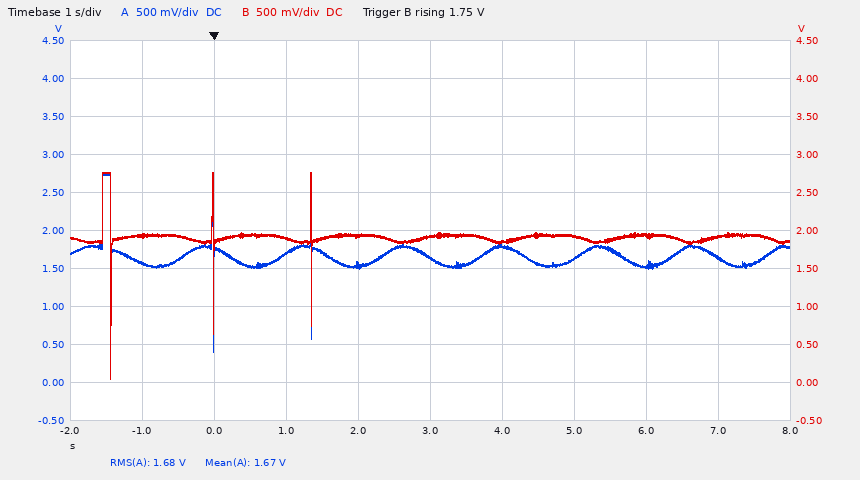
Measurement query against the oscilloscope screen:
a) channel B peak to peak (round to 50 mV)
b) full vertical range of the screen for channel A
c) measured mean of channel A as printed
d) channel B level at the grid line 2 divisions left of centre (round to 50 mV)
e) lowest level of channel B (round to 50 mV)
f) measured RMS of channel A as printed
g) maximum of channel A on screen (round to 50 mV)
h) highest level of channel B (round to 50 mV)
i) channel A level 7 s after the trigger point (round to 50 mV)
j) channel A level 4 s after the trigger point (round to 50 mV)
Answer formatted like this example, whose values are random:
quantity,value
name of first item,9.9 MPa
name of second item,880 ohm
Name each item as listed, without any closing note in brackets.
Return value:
quantity,value
channel B peak to peak,2.70 V
full vertical range of the screen for channel A,5 V
measured mean of channel A as printed,1.67 V
channel B level at the grid line 2 divisions left of centre,1.90 V
lowest level of channel B,50 mV
measured RMS of channel A as printed,1.68 V
maximum of channel A on screen,2.75 V
highest level of channel B,2.75 V
channel A level 7 s after the trigger point,1.65 V
channel A level 4 s after the trigger point,1.80 V
